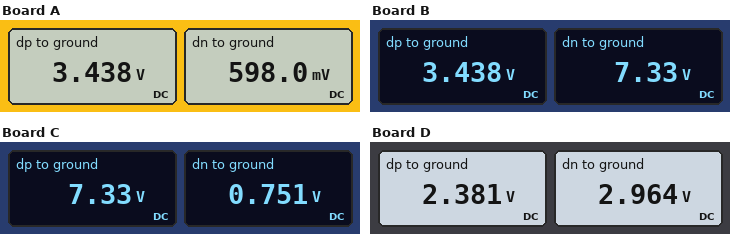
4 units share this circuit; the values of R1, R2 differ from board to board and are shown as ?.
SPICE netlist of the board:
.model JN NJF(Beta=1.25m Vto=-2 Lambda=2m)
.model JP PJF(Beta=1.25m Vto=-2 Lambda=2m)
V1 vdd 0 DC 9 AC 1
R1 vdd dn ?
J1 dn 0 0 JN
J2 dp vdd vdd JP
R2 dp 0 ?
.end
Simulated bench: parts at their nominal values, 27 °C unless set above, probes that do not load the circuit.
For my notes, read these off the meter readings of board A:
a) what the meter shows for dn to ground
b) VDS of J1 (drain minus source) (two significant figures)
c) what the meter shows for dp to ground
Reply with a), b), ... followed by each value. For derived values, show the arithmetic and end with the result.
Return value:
a) 598.0 mV
b) 598 mV = 600 mV
c) 3.438 V
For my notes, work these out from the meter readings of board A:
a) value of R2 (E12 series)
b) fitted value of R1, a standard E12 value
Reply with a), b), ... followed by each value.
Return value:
a) 680 Ω
b) 3.3 kΩ
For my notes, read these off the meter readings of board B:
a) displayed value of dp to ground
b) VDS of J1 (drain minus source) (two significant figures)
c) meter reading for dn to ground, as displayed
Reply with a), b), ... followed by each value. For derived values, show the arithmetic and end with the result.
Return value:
a) 3.438 V
b) 7.33 V = 7.3 V
c) 7.33 V
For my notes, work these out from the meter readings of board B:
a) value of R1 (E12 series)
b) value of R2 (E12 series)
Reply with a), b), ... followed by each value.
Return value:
a) 330 Ω
b) 680 Ω
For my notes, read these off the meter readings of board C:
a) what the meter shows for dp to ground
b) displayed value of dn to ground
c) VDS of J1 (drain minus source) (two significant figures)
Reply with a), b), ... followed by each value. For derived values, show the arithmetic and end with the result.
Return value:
a) 7.33 V
b) 0.751 V
c) 751 mV = 750 mV
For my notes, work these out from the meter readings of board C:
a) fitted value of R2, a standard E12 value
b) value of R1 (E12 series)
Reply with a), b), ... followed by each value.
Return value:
a) 1.5 kΩ
b) 2.7 kΩ
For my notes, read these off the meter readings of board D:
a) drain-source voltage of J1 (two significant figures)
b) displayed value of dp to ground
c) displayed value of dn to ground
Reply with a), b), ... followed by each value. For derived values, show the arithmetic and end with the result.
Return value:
a) 2.964 V = 3.0 V
b) 2.381 V
c) 2.964 V
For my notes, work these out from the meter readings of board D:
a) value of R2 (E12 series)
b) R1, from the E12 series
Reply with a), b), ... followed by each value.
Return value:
a) 470 Ω
b) 1.2 kΩ
